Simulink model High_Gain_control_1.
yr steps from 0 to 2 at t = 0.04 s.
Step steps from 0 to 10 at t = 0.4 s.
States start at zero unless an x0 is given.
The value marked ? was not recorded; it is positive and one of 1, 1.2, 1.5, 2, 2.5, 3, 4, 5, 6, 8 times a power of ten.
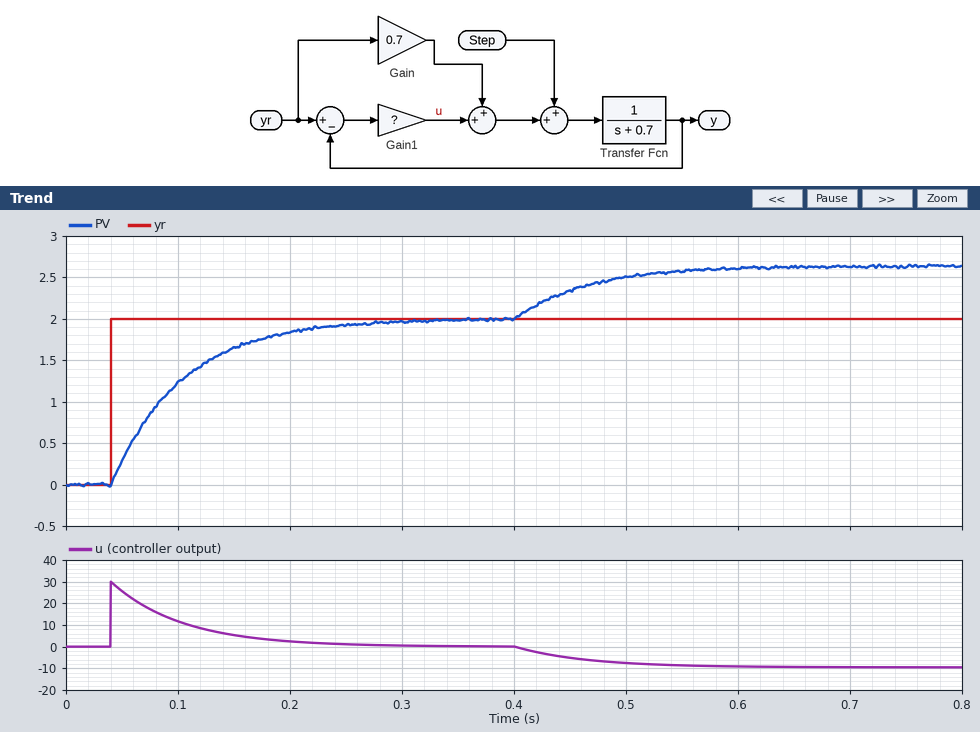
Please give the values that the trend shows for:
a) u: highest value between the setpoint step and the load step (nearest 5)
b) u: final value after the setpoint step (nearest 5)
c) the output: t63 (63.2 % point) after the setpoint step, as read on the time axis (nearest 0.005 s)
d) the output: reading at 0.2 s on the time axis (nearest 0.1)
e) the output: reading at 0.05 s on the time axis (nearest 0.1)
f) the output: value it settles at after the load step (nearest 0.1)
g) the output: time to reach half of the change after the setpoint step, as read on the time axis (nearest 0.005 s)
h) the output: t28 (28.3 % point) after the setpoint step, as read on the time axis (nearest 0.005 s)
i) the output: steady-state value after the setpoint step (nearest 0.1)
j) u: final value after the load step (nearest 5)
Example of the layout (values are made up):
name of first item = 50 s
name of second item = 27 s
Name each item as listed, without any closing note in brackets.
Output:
u: highest value between the setpoint step and the load step = 30
u: final value after the setpoint step = 0
the output: t63 (63.2 % point) after the setpoint step, as read on the time axis = 0.105 s
the output: reading at 0.2 s on the time axis = 1.8
the output: reading at 0.05 s on the time axis = 0.3
the output: value it settles at after the load step = 2.6
the output: time to reach half of the change after the setpoint step, as read on the time axis = 0.085 s
the output: t28 (28.3 % point) after the setpoint step, as read on the time axis = 0.060 s
the output: steady-state value after the setpoint step = 2.0
u: final value after the load step = -10
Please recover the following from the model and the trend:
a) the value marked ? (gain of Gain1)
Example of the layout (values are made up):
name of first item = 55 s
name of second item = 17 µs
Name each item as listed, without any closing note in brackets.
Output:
the value marked ? = 15
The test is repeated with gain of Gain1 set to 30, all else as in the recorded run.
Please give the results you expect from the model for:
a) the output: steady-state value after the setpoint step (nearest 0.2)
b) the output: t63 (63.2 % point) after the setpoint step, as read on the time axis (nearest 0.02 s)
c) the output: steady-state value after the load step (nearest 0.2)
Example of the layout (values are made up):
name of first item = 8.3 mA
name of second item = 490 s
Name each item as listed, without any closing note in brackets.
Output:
the output: steady-state value after the setpoint step = 2.0
the output: t63 (63.2 % point) after the setpoint step, as read on the time axis = 0.08 s
the output: steady-state value after the load step = 2.4
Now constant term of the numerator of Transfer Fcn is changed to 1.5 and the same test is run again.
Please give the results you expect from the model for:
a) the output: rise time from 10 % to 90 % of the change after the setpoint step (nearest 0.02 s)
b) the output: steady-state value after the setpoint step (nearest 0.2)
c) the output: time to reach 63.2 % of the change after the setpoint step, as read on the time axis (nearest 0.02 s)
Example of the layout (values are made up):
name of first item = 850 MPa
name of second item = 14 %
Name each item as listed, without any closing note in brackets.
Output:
the output: rise time from 10 % to 90 % of the change after the setpoint step = 0.10 s
the output: steady-state value after the setpoint step = 2.0
the output: time to reach 63.2 % of the change after the setpoint step, as read on the time axis = 0.08 s
